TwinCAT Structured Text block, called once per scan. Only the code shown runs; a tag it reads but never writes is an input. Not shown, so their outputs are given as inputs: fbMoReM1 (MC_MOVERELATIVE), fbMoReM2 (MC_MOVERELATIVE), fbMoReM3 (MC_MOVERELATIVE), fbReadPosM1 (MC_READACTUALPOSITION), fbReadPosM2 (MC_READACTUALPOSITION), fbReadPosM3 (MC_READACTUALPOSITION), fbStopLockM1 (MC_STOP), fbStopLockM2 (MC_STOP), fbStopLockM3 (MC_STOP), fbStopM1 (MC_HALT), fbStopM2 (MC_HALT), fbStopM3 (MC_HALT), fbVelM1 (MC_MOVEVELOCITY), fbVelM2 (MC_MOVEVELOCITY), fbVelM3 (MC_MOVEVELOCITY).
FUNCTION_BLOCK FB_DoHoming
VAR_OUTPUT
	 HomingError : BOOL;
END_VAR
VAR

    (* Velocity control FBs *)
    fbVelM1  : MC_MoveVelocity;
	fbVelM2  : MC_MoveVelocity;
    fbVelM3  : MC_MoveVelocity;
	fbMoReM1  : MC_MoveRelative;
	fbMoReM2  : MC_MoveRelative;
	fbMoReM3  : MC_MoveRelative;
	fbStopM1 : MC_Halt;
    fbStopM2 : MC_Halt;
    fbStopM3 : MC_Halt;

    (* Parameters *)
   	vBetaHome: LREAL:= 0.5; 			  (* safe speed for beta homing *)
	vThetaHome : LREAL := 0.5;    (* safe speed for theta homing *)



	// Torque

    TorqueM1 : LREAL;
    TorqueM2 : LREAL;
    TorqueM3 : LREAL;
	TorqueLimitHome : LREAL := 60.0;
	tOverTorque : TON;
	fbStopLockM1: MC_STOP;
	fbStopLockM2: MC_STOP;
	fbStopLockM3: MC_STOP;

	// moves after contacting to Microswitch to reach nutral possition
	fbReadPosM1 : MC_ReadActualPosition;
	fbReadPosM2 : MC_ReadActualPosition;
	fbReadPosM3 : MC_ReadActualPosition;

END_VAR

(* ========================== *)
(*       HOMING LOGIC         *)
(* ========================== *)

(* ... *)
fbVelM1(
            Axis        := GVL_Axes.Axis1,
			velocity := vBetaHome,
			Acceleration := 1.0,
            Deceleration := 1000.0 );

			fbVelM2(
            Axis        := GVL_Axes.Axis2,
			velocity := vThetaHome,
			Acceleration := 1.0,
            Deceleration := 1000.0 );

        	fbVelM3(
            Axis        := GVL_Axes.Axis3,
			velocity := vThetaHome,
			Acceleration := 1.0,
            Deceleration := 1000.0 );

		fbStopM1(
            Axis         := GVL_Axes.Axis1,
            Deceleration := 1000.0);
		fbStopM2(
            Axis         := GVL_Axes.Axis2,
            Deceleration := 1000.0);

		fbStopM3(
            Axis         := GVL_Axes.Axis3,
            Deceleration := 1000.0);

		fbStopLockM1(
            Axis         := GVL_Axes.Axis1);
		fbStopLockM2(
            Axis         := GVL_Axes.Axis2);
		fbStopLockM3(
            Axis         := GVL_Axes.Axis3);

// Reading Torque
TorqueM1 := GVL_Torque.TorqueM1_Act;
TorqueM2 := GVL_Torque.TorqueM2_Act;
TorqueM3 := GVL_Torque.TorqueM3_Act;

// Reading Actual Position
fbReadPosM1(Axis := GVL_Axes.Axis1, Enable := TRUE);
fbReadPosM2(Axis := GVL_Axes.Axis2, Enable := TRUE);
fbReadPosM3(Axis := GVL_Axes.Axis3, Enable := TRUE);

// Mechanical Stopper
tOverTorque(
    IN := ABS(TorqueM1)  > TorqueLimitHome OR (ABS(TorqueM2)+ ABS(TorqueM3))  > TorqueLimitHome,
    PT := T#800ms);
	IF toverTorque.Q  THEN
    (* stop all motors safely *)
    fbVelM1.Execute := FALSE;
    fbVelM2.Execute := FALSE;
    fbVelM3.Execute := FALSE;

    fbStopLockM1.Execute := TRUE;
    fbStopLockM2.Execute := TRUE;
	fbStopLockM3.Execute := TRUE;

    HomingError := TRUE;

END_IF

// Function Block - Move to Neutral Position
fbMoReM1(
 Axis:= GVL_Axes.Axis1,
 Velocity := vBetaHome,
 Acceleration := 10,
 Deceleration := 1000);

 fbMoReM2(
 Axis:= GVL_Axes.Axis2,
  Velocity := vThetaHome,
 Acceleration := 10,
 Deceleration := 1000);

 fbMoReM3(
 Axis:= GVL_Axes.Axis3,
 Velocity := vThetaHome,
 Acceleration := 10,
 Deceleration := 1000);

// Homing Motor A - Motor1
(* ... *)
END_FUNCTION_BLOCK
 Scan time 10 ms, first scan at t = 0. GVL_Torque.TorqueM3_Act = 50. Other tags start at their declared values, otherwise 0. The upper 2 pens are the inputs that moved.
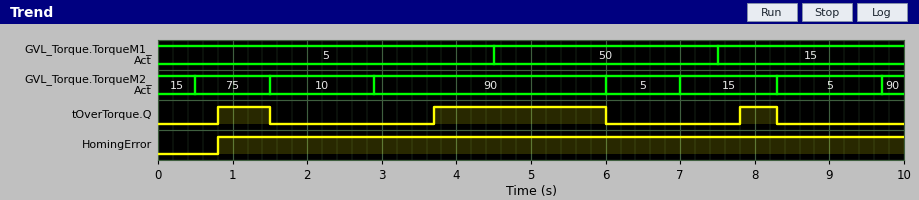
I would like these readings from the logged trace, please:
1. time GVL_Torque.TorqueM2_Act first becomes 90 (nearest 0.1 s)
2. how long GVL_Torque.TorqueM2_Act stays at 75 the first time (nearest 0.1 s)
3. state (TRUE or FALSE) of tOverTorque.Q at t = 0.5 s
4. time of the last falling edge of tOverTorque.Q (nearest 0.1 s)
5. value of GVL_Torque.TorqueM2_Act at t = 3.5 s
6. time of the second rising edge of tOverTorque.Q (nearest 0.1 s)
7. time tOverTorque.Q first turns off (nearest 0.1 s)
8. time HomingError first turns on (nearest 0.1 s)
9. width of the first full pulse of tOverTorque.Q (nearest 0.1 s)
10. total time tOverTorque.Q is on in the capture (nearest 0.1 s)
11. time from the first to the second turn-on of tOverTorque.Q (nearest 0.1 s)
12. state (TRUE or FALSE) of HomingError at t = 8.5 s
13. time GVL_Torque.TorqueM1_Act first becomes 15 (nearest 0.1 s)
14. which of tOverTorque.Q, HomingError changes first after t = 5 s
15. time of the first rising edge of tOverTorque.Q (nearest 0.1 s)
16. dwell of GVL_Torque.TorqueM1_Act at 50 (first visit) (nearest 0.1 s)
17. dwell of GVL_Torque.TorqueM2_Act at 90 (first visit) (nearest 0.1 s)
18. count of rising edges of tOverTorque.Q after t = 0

2.9 s
1.0 s
FALSE
8.3 s
90
3.7 s
1.5 s
0.8 s
0.7 s
3.5 s
2.9 s
TRUE
7.5 s
tOverTorque.Q
0.8 s
3.0 s
3.1 s
3
